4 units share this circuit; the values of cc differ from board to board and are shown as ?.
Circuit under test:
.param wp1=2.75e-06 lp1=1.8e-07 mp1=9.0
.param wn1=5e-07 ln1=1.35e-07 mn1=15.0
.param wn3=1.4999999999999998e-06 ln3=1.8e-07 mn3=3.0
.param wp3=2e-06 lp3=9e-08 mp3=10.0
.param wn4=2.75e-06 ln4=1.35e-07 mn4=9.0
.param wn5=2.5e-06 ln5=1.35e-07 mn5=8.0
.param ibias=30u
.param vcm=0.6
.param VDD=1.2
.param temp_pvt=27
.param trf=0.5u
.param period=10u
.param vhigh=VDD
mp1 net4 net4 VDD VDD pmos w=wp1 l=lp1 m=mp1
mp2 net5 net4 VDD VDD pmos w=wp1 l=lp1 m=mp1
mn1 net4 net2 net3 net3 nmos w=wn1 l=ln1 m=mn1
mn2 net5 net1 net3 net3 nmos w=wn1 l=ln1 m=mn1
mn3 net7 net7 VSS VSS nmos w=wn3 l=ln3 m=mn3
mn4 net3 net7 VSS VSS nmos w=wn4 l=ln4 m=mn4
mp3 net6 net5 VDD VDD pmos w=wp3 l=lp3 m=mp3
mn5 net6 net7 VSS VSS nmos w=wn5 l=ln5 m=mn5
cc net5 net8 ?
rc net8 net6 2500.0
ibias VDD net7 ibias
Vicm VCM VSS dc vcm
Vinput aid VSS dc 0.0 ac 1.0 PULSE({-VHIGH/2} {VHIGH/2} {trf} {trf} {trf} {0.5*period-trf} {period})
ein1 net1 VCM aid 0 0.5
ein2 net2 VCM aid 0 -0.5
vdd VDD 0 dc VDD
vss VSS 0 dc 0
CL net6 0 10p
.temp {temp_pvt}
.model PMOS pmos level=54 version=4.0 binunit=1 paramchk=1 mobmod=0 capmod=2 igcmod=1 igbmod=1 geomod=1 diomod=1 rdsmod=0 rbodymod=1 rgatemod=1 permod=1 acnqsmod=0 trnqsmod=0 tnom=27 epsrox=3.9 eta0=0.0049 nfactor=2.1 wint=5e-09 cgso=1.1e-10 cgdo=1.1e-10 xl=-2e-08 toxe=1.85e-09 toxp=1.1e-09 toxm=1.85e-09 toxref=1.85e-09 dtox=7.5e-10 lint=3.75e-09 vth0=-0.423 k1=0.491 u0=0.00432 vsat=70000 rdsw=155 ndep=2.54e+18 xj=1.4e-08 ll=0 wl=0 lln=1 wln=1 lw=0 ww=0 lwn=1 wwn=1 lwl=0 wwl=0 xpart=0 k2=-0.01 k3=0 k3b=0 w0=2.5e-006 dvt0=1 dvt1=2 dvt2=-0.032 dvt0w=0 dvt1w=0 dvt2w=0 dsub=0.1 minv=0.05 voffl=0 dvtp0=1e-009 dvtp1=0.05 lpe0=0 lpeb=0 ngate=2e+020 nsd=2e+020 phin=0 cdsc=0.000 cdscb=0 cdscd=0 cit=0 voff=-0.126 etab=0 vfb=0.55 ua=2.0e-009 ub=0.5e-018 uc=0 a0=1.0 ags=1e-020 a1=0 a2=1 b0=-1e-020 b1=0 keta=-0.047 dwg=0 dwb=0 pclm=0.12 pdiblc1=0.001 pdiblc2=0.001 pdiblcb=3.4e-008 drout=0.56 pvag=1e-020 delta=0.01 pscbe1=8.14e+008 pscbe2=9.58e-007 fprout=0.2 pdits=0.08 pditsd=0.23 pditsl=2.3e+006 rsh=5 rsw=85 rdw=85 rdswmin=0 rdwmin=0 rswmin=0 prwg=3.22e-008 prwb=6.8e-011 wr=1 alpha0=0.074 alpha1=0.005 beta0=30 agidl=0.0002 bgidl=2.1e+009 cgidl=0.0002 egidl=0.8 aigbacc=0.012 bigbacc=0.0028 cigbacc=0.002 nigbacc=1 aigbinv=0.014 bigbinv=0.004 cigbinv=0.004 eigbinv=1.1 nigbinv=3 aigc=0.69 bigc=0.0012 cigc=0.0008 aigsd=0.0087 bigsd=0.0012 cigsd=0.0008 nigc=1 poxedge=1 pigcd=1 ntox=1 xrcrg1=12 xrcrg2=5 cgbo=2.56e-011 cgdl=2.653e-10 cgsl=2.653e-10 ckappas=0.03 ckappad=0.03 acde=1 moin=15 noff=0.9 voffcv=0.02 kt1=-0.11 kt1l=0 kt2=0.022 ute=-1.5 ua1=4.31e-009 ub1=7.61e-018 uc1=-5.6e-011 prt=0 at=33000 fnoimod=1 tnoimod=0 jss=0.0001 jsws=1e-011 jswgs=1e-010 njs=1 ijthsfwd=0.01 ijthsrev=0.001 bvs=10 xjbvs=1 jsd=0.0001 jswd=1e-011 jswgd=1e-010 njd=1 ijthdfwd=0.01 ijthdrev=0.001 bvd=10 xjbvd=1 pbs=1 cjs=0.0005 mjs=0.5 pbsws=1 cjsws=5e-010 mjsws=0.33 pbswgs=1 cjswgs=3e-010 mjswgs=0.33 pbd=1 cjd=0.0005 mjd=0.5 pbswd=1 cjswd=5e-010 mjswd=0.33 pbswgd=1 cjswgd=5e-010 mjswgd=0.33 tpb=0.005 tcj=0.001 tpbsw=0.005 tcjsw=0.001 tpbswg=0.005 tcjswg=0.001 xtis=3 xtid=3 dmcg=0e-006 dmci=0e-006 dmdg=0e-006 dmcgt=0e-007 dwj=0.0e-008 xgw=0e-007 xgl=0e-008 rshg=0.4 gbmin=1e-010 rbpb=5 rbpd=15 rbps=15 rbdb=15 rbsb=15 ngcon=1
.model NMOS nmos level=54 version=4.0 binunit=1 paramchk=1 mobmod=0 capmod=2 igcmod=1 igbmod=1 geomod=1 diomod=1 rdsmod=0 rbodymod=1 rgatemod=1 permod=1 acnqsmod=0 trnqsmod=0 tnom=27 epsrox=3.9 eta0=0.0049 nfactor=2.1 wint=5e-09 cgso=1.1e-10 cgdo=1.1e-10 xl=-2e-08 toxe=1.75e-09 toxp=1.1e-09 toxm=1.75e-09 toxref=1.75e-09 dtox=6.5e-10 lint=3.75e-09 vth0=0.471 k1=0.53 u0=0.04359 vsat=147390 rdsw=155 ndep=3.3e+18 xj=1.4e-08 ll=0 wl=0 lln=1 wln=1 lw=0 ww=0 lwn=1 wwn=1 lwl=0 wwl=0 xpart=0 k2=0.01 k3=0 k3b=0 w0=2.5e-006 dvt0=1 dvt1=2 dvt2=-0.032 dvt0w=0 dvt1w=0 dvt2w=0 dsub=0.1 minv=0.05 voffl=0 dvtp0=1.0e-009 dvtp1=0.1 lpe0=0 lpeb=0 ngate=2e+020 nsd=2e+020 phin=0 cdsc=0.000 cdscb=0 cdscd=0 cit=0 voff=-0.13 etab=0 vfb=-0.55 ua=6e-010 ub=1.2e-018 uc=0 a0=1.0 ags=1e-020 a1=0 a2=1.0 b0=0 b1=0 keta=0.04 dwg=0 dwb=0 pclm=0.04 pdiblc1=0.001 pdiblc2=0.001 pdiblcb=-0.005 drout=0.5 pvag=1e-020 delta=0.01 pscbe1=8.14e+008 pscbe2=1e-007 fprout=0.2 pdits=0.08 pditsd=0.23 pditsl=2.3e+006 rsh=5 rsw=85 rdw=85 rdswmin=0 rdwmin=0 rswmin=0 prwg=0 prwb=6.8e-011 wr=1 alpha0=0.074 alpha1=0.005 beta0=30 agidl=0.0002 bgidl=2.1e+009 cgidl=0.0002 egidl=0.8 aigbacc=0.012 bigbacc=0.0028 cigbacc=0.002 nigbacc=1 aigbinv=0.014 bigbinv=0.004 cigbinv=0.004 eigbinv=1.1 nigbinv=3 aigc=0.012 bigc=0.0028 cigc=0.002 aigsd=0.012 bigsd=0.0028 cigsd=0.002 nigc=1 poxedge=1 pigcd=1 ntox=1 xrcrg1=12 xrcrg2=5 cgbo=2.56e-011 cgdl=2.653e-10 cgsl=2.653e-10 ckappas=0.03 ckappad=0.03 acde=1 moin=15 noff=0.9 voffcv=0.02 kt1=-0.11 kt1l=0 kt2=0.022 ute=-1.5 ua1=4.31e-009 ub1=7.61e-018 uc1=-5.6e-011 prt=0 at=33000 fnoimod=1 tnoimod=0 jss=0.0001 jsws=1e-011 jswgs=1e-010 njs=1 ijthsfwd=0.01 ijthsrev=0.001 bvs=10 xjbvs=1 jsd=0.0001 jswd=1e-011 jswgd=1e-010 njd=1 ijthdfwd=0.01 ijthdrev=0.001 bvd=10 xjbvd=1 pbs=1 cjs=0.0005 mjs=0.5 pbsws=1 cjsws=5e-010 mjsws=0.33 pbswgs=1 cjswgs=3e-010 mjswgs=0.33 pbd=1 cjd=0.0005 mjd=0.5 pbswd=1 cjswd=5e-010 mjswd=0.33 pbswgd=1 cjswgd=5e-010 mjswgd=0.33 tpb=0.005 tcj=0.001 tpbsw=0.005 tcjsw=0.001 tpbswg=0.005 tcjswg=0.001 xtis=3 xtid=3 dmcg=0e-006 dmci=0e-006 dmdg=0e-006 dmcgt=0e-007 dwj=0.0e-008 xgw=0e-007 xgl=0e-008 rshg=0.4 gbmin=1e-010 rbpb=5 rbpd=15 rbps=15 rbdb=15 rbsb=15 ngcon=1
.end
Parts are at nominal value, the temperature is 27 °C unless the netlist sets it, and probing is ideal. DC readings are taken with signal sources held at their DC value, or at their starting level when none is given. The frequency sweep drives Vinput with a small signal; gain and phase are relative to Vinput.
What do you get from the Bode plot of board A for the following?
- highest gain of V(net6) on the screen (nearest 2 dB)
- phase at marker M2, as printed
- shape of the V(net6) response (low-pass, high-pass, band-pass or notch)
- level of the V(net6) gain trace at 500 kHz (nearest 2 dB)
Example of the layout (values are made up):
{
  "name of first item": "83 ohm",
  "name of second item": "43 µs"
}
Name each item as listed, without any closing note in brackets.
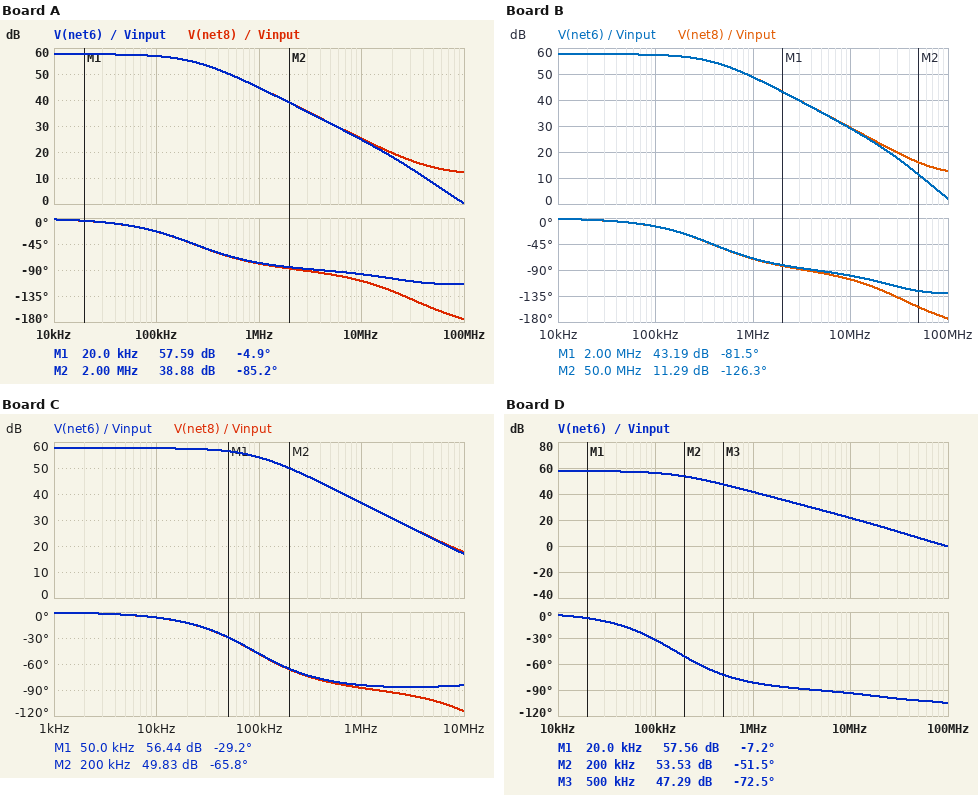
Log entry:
{
  "highest gain of V(net6) on the screen": "58 dB",
  "phase at marker M2, as printed": "-85.2 deg",
  "shape of the V(net6) response": "low-pass",
  "level of the V(net6) gain trace at 500 kHz": "50 dB"
}
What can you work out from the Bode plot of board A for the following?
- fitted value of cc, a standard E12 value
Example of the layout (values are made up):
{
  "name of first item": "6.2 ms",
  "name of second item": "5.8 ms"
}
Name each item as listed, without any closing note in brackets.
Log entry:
{
  "fitted value of cc, a standard E12 value": "1.2 pF"
}
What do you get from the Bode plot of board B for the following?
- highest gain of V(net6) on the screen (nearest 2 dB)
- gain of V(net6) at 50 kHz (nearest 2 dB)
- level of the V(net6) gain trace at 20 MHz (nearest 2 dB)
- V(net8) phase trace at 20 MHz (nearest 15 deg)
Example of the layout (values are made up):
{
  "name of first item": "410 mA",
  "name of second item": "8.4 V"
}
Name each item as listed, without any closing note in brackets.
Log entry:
{
  "highest gain of V(net6) on the screen": "58 dB",
  "gain of V(net6) at 50 kHz": "58 dB",
  "level of the V(net6) gain trace at 20 MHz": "22 dB",
  "V(net8) phase trace at 20 MHz": "-120 deg"
}
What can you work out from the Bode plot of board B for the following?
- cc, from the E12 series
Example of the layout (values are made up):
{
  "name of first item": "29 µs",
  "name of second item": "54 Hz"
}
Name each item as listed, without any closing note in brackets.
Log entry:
{
  "cc, from the E12 series": "680 fF"
}
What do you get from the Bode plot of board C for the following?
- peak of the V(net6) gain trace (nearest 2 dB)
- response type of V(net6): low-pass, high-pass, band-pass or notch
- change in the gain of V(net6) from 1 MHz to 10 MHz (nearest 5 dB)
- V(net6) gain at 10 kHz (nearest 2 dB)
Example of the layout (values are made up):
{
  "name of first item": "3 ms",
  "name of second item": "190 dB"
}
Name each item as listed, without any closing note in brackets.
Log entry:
{
  "peak of the V(net6) gain trace": "58 dB",
  "response type of V(net6): low-pass, high-pass, band-pass or notch": "low-pass",
  "change in the gain of V(net6) from 1 MHz to 10 MHz": "-20 dB",
  "V(net6) gain at 10 kHz": "58 dB"
}
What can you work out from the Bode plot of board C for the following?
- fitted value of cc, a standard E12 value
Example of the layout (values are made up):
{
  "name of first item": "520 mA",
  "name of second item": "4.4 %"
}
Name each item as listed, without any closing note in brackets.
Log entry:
{
  "fitted value of cc, a standard E12 value": "3.3 pF"
}
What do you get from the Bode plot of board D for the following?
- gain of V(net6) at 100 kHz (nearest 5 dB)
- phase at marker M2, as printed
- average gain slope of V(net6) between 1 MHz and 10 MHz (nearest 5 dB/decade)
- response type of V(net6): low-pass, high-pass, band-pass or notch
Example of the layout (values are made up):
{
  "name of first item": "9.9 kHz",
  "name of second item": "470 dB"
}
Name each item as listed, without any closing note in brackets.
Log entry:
{
  "gain of V(net6) at 100 kHz": "55 dB",
  "phase at marker M2, as printed": "-51.5 deg",
  "average gain slope of V(net6) between 1 MHz and 10 MHz": "-20 dB/decade",
  "response type of V(net6): low-pass, high-pass, band-pass or notch": "low-pass"
}
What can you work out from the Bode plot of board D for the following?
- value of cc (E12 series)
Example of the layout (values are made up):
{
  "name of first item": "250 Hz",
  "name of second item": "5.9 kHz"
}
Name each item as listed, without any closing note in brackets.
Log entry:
{
  "value of cc": "1.8 pF"
}
